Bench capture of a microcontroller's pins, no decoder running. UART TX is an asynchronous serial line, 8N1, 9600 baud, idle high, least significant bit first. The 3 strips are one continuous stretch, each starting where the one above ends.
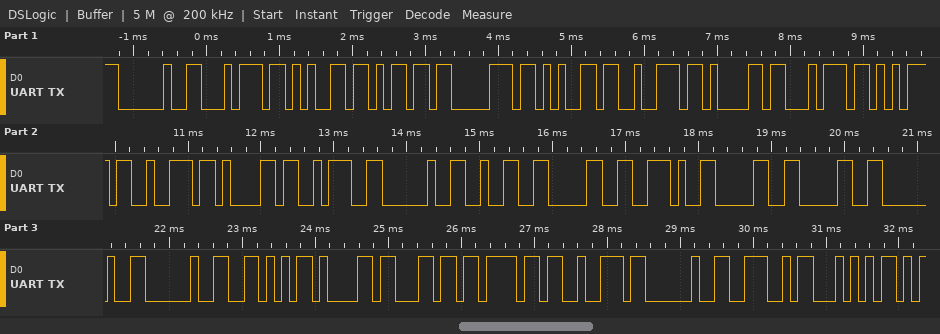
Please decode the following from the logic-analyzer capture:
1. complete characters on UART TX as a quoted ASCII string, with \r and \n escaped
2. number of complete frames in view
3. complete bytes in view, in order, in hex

" temperatura: 20.00  Valor NT"
29
0x20 0x74 0x65 0x6D 0x70 0x65 0x72 0x61 0x74 0x75 0x72 0x61 0x3A 0x20 0x32 0x30 0x2E 0x30 0x30 0x20 0x20 0x56 0x61 0x6C 0x6F 0x72 0x20 0x4E 0x54
